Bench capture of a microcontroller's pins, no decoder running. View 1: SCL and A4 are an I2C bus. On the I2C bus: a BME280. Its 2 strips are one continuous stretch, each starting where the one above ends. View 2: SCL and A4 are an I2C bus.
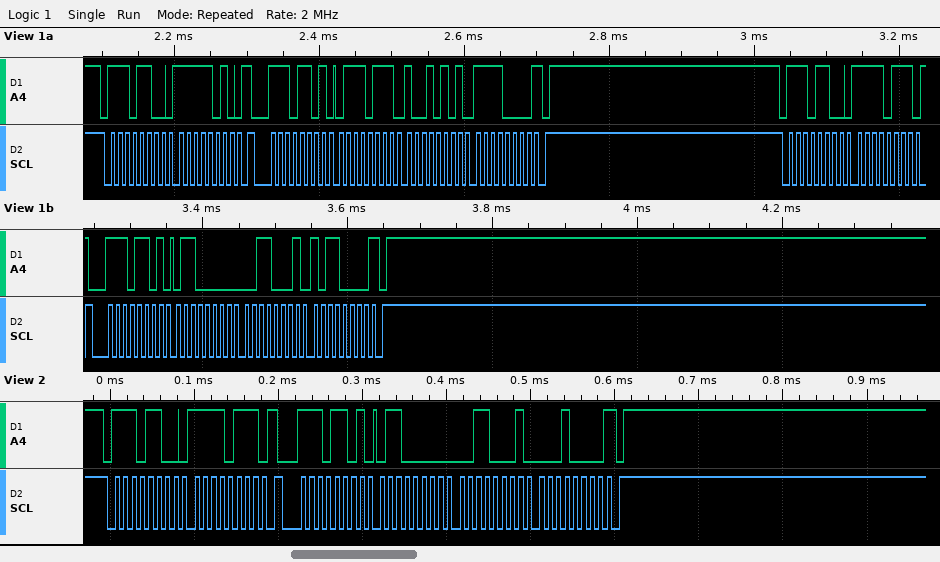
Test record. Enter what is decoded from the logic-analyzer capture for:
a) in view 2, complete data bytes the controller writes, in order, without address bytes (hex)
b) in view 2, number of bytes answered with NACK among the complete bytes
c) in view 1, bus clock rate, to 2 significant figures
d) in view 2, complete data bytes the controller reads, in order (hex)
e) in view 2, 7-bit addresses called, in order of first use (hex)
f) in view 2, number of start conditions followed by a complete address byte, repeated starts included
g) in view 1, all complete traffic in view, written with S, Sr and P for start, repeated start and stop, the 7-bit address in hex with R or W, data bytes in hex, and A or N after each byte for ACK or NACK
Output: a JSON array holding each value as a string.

["F7", "1", "100 kHz", "60 31 10", "0x76", "2", "S 76W A FA A Sr 76R A 77 A 95 A F0 N P S 76W A F7 A Sr 76R A 60 A 31 A B0 N P"]
